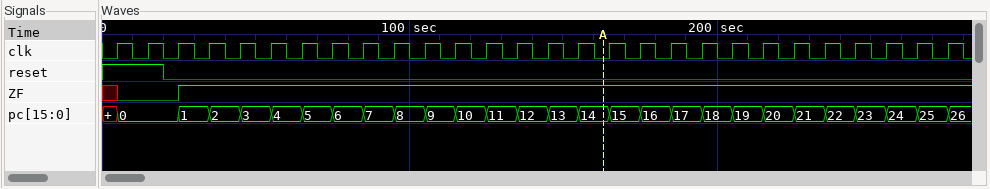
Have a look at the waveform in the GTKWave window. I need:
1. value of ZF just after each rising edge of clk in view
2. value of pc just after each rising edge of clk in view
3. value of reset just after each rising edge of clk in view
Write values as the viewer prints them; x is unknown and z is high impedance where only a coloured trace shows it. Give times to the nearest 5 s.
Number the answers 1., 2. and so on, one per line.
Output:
1. 0 0 1 1 1 1 1 1 1 1 1 1 1 1 1 1 1 1 1 1 1 1 1 1 1 1 1 1
2. 0, 0, 1, 2, 3, 4, 5, 6, 7, 8, 9, 10, 11, 12, 13, 14, 15, 16, 17, 18, 19, 20, 21, 22, 23, 24, 25, 26
3. 1 1 0 0 0 0 0 0 0 0 0 0 0 0 0 0 0 0 0 0 0 0 0 0 0 0 0 0
